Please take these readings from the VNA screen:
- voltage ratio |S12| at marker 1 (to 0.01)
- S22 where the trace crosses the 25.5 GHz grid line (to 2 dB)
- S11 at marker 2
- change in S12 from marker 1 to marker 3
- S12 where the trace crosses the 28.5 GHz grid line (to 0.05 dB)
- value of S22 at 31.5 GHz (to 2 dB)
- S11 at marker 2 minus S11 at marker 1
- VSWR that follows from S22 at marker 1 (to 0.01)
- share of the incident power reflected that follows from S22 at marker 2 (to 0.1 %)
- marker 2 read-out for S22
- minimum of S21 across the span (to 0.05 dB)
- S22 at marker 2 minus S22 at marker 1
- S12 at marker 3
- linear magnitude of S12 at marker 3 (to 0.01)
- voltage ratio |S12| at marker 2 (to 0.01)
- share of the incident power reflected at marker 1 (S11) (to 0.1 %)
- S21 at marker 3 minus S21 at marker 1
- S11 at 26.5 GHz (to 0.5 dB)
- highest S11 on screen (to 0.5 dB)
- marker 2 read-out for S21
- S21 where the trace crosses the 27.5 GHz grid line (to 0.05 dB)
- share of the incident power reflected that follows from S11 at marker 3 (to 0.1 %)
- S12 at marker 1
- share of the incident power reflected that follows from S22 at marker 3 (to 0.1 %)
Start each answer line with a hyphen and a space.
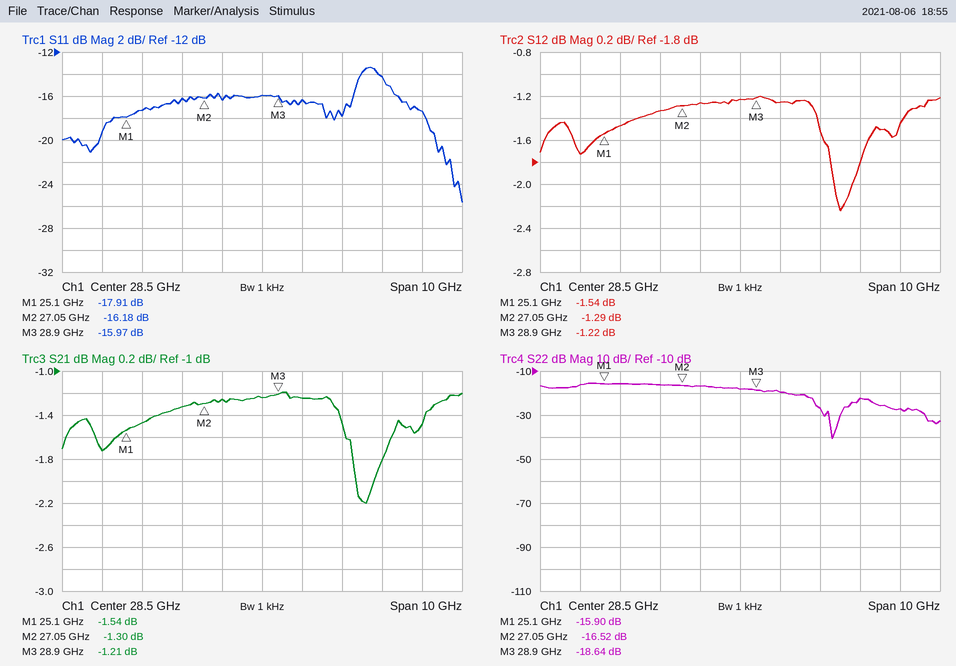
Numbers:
- 0.84
- -16 dB
- -16.18 dB
- 0.32 dB
- -1.25 dB
- -22 dB
- 1.73 dB
- 1.38
- 2.2 %
- -16.52 dB
- -2.20 dB
- -0.62 dB
- -1.22 dB
- 0.87
- 0.86
- 1.6 %
- 0.33 dB
- -16.0 dB
- -13.5 dB
- -1.30 dB
- -1.25 dB
- 2.5 %
- -1.54 dB
- 1.4 %
